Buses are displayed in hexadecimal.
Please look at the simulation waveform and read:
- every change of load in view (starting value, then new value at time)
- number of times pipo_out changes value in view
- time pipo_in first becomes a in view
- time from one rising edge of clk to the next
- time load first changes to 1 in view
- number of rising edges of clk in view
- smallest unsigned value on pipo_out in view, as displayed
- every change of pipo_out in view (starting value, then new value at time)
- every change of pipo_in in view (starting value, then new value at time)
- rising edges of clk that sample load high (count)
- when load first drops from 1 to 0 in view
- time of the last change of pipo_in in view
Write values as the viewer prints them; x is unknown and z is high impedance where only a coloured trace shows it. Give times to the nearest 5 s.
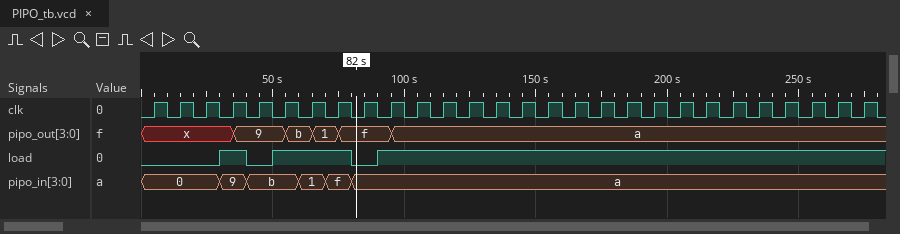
0, 1 at 30 s, 0 at 40 s, 1 at 50 s, 0 at 80 s, 1 at 90 s
5
80 s
10 s
30 s
28
1
x, 9 at 35 s, b at 55 s, 1 at 65 s, f at 75 s, a at 95 s
0, 9 at 30 s, b at 40 s, 1 at 60 s, f at 70 s, a at 80 s
23
40 s
80 s
